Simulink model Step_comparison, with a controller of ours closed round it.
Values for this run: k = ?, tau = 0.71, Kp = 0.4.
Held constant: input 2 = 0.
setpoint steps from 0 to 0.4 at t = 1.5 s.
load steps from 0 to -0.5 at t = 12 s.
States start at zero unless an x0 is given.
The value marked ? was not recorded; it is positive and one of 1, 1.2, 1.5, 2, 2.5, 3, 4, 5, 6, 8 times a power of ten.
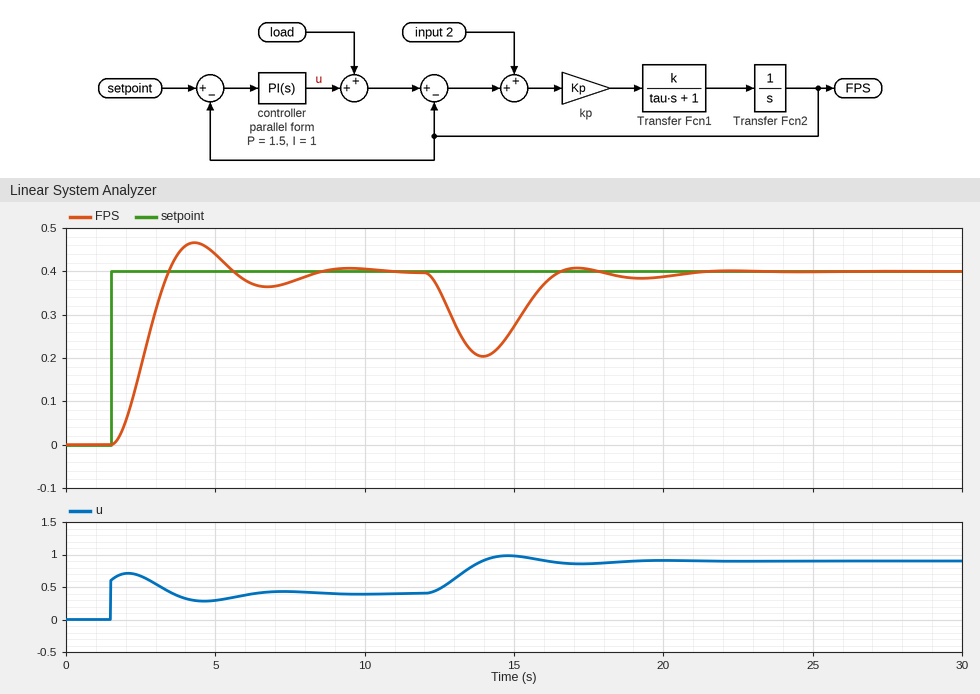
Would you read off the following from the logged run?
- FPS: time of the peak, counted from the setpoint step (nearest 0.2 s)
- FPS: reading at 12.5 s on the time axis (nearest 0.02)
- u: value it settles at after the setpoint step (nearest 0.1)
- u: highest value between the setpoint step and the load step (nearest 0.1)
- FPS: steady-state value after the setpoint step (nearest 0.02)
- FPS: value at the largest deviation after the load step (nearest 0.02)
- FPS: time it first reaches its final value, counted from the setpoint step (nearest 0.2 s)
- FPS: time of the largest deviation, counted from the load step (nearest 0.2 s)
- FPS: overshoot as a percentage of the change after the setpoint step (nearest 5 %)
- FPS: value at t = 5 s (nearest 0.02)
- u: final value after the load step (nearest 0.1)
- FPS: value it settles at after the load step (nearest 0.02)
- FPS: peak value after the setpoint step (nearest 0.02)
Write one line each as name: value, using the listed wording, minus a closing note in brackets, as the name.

FPS: time of the peak, counted from the setpoint step: 2.8 s
FPS: reading at 12.5 s on the time axis: 0.36
u: value it settles at after the setpoint step: 0.4
u: highest value between the setpoint step and the load step: 0.7
FPS: steady-state value after the setpoint step: 0.40
FPS: value at the largest deviation after the load step: 0.20
FPS: time it first reaches its final value, counted from the setpoint step: 2.0 s
FPS: time of the largest deviation, counted from the load step: 2.0 s
FPS: overshoot as a percentage of the change after the setpoint step: 15 %
FPS: value at t = 5 s: 0.44
u: final value after the load step: 0.9
FPS: value it settles at after the load step: 0.40
FPS: peak value after the setpoint step: 0.46
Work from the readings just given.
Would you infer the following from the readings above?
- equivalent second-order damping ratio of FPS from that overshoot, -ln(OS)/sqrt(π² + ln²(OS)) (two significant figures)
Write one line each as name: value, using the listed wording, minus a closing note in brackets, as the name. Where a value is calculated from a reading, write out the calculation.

equivalent second-order damping ratio of FPS from that overshoot, -ln(OS)/sqrt(π² + ln²(OS)): ln(0.15) = -1.897; 1.897 / sqrt(9.870 + 3.599) = 0.52
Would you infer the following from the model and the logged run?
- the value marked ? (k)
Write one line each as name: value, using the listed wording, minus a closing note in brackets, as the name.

the value marked ?: 1.5
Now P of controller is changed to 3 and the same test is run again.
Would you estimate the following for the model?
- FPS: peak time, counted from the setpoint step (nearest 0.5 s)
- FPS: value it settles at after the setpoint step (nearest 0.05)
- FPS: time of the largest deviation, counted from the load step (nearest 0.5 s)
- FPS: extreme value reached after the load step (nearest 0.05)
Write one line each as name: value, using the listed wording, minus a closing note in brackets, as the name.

FPS: peak time, counted from the setpoint step: 2.0 s
FPS: value it settles at after the setpoint step: 0.40
FPS: time of the largest deviation, counted from the load step: 1.5 s
FPS: extreme value reached after the load step: 0.25
